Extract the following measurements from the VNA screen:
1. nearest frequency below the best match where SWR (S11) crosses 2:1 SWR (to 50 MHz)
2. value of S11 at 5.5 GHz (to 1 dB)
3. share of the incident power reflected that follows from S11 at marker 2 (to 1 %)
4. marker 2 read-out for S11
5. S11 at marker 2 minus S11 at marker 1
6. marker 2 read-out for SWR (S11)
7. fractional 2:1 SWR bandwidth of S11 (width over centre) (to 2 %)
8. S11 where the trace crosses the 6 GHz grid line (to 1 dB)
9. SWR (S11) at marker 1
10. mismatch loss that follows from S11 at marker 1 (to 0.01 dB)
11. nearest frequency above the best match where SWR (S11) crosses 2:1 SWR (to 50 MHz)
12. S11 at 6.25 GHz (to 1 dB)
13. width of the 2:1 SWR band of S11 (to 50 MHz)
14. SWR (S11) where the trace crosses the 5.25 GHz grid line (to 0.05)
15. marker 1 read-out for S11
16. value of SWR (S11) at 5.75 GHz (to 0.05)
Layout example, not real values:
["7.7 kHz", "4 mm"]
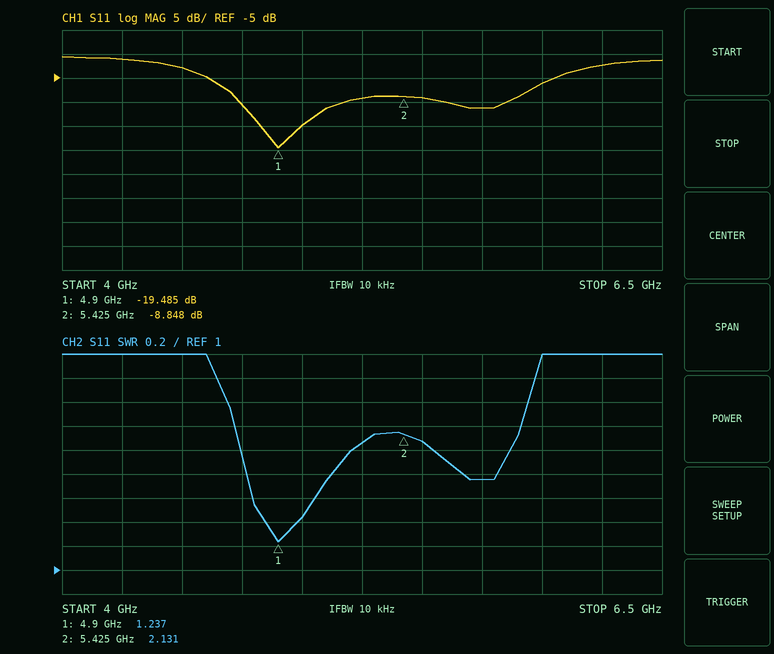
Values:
["4.75 GHz", "-9 dB", "13 %", "-8.848 dB", "10.637 dB", "2.131", "10 %", "-6 dB", "1.237", "0.05 dB", "5.20 GHz", "-2 dB", "450 MHz", "2.05", "-19.485 dB", "1.75"]
